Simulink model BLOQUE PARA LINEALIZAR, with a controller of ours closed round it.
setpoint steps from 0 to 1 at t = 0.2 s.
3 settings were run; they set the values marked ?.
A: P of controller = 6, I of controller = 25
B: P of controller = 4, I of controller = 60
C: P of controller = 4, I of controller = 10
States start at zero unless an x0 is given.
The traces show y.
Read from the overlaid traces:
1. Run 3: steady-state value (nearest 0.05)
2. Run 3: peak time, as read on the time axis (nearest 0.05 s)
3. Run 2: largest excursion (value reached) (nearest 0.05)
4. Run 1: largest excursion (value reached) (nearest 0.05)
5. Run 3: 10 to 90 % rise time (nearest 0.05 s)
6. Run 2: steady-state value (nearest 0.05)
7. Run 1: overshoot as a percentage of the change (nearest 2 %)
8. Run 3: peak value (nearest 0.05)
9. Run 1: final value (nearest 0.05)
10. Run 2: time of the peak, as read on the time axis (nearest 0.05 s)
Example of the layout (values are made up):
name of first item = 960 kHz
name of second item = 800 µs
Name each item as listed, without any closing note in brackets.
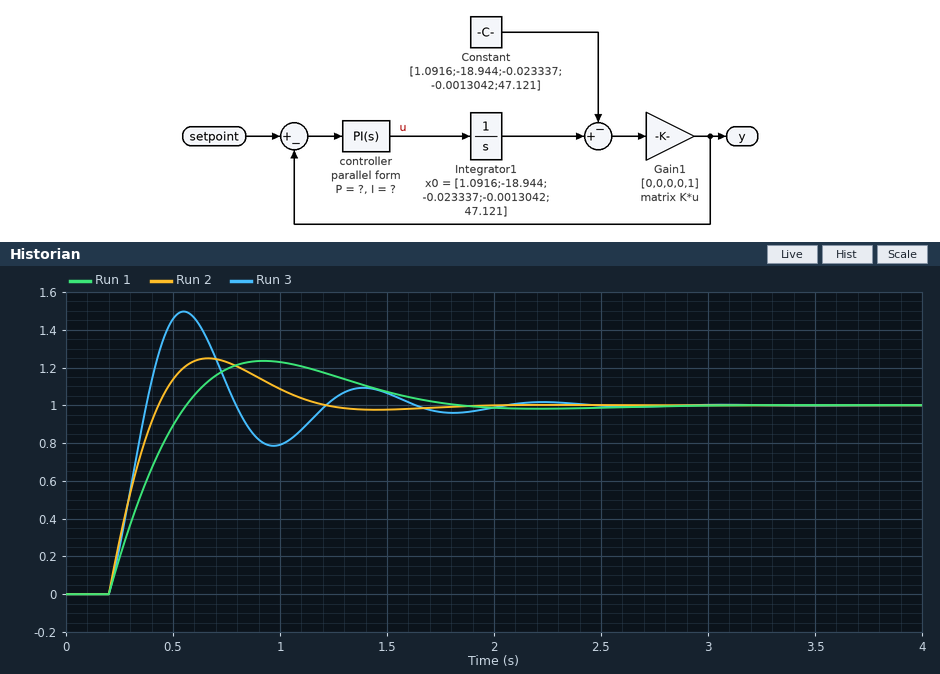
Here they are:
Run 3: steady-state value = 1.00
Run 3: peak time, as read on the time axis = 0.55 s
Run 2: largest excursion (value reached) = 1.25
Run 1: largest excursion (value reached) = 1.25
Run 3: 10 to 90 % rise time = 0.15 s
Run 2: steady-state value = 1.00
Run 1: overshoot as a percentage of the change = 24 %
Run 3: peak value = 1.50
Run 1: final value = 1.00
Run 2: time of the peak, as read on the time axis = 0.65 s
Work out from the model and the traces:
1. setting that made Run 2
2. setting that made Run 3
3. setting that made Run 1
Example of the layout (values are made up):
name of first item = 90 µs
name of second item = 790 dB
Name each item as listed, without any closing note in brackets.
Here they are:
setting that made Run 2 = A
setting that made Run 3 = B
setting that made Run 1 = C
